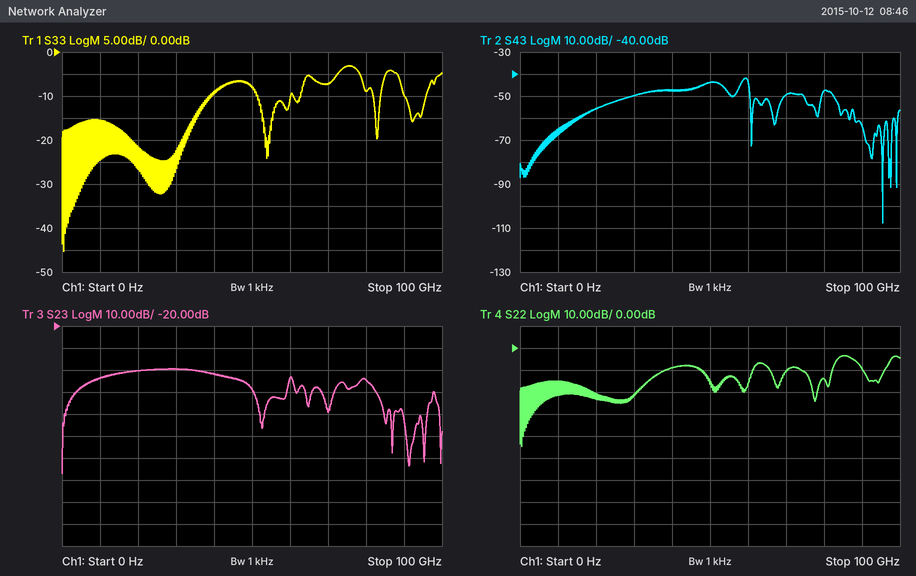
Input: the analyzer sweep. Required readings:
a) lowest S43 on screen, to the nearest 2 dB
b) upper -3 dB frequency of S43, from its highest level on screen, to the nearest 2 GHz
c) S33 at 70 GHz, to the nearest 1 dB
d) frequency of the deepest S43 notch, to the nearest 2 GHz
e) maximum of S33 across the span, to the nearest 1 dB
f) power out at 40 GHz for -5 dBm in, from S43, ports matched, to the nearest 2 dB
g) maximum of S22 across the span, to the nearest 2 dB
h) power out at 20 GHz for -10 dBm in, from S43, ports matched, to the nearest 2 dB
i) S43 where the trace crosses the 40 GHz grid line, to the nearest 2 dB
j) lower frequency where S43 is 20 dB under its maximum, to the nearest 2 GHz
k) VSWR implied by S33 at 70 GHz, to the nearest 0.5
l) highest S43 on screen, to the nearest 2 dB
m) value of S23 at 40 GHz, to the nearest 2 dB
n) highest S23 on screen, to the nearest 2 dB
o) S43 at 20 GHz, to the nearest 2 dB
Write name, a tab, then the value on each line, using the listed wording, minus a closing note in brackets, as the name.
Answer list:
lowest S43 on screen, to the nearest 2 dB	-108 dB
upper -3 dB frequency of S43, from its highest level on screen, to the nearest 2 GHz	60 GHz
S33 at 70 GHz, to the nearest 1 dB	-7 dB
frequency of the deepest S43 notch, to the nearest 2 GHz	96 GHz
maximum of S33 across the span, to the nearest 1 dB	-3 dB
power out at 40 GHz for -5 dBm in, from S43, ports matched, to the nearest 2 dB	-52 dBm
maximum of S22 across the span, to the nearest 2 dB	-4 dB
power out at 20 GHz for -10 dBm in, from S43, ports matched, to the nearest 2 dB	-66 dBm
S43 where the trace crosses the 40 GHz grid line, to the nearest 2 dB	-48 dB
lower frequency where S43 is 20 dB under its maximum, to the nearest 2 GHz	14 GHz
VSWR implied by S33 at 70 GHz, to the nearest 0.5	2.5
highest S43 on screen, to the nearest 2 dB	-42 dB
value of S23 at 40 GHz, to the nearest 2 dB	-42 dB
highest S23 on screen, to the nearest 2 dB	-40 dB
S43 at 20 GHz, to the nearest 2 dB	-56 dB
